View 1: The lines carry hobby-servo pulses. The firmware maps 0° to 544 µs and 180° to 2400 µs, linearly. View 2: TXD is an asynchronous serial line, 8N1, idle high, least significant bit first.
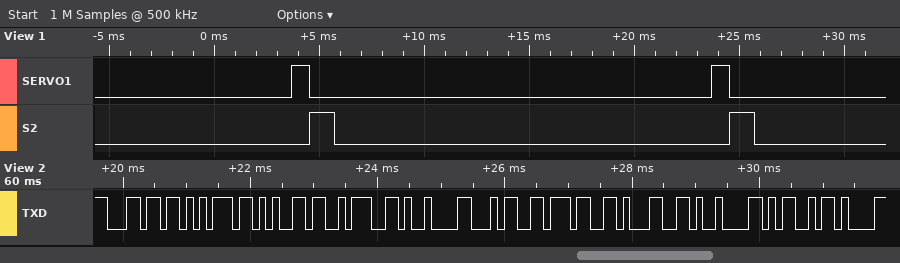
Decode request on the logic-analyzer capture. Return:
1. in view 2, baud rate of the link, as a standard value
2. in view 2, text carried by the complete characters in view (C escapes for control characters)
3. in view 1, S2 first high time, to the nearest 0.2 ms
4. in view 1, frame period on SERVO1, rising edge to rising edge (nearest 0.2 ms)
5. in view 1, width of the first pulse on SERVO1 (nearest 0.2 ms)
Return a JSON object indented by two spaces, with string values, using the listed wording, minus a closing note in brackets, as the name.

{
  "in view 2, baud rate of the link, as a standard value": "9600 baud",
  "in view 2, text carried by the complete characters in view": "\"lue:\\t471\\tM\"",
  "in view 1, S2 first high time, to the nearest 0.2 ms": "1.2 ms",
  "in view 1, frame period on SERVO1, rising edge to rising edge": "20.0 ms",
  "in view 1, width of the first pulse on SERVO1": "0.8 ms"
}
